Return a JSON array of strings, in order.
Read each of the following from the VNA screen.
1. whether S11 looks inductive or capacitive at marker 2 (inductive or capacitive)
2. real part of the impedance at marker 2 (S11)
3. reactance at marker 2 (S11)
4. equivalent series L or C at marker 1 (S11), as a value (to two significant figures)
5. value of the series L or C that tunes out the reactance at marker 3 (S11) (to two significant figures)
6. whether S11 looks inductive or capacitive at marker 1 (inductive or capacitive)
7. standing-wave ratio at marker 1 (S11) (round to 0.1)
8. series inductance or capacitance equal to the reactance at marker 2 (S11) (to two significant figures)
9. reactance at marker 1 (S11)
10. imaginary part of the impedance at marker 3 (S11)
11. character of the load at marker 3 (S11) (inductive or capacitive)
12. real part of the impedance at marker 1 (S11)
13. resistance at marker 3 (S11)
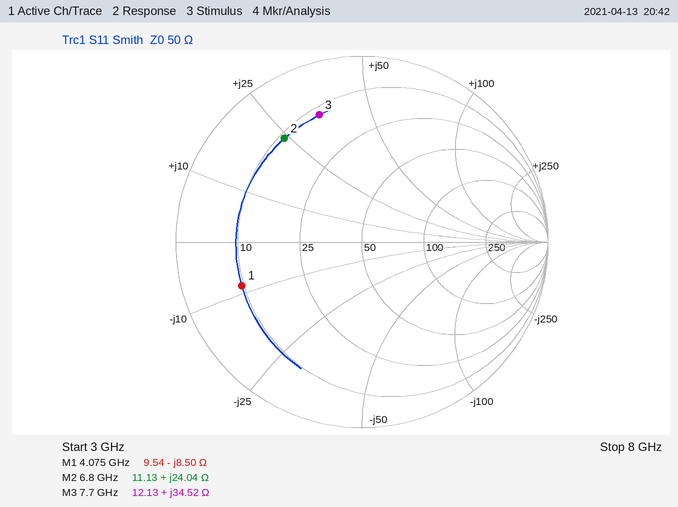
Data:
["inductive", "11.13 Ω", "+24.04 Ω", "4.6 pF", "600 fF", "capacitive", "5.4", "560 pH", "-8.50 Ω", "+34.52 Ω", "inductive", "9.54 Ω", "12.13 Ω"]
